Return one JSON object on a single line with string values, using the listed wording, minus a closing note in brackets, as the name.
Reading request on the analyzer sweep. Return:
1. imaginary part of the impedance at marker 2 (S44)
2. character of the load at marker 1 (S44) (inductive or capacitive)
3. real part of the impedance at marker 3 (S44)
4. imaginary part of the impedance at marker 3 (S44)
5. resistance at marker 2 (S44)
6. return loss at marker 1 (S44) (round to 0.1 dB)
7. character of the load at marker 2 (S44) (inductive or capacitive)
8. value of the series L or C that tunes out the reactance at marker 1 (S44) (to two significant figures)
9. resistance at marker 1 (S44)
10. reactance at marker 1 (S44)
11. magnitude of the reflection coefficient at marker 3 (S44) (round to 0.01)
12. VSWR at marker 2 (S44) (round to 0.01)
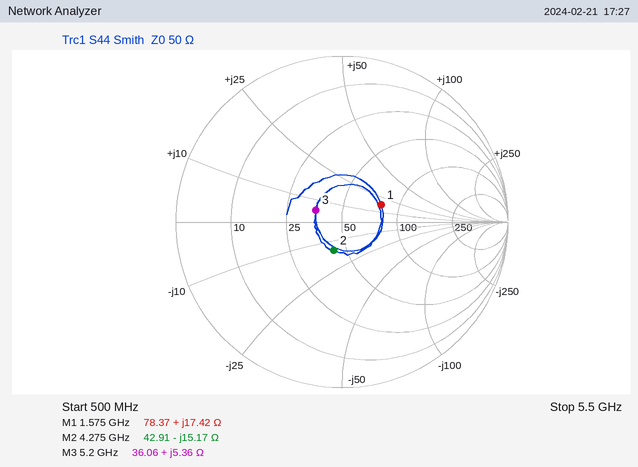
{"imaginary part of the impedance at marker 2": "-15.17 Ω", "character of the load at marker 1 (S44)": "inductive", "real part of the impedance at marker 3": "36.06 Ω", "imaginary part of the impedance at marker 3": "+5.36 Ω", "resistance at marker 2": "42.91 Ω", "return loss at marker 1 (S44)": "11.8 dB", "character of the load at marker 2 (S44)": "capacitive", "value of the series L or C that tunes out the reactance at marker 1 (S44)": "5.8 pF", "resistance at marker 1": "78.37 Ω", "reactance at marker 1": "+17.42 Ω", "magnitude of the reflection coefficient at marker 3 (S44)": "0.17", "VSWR at marker 2 (S44)": "1.43"}
